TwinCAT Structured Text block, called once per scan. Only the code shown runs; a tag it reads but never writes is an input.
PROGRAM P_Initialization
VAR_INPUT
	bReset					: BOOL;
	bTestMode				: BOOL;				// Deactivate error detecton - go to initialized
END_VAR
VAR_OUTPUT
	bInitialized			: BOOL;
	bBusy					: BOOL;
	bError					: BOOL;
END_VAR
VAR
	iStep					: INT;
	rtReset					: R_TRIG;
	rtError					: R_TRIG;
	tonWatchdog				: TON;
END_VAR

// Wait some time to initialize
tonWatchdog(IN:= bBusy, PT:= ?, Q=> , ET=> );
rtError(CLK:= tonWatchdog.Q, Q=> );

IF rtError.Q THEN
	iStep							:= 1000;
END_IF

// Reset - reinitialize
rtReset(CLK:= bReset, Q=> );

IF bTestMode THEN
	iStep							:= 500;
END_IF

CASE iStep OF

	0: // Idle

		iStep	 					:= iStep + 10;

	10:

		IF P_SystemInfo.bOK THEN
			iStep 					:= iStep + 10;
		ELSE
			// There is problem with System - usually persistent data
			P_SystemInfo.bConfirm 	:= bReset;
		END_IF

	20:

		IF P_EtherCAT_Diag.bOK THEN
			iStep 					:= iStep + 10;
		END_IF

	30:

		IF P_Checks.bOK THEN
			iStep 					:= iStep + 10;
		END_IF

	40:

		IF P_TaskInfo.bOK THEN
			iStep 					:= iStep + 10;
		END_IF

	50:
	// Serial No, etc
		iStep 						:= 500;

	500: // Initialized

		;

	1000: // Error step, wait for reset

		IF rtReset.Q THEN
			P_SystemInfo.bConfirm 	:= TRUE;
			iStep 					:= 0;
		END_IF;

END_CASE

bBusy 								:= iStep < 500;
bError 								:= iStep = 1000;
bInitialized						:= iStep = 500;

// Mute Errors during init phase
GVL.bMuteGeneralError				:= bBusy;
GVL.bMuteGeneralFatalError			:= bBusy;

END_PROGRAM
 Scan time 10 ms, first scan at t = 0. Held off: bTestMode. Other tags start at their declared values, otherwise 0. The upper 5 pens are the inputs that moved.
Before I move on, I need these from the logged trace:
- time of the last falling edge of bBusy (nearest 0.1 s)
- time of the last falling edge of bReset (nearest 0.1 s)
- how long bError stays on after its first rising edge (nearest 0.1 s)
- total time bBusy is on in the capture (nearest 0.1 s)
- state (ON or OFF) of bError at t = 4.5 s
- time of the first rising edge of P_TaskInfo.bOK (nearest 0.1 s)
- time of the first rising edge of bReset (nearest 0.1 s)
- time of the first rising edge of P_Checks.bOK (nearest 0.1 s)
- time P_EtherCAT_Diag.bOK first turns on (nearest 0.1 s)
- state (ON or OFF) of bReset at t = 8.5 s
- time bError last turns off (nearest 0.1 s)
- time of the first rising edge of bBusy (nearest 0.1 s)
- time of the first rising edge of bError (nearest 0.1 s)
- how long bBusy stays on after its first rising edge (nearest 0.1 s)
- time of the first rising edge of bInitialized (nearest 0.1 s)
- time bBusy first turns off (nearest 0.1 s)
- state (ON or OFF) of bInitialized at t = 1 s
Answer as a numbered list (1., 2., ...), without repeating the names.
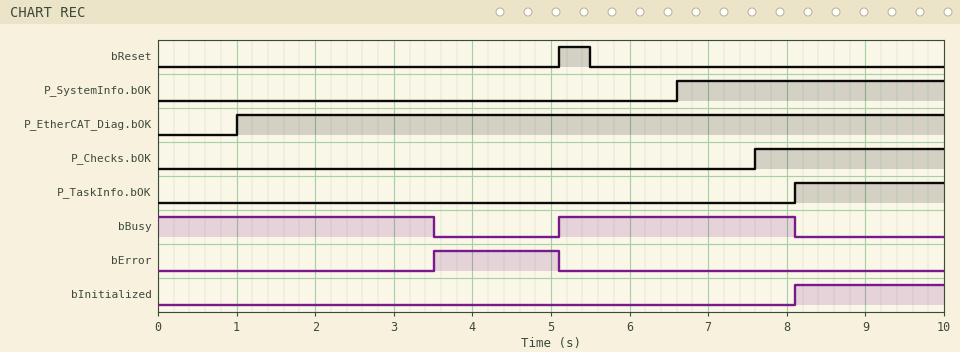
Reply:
1. 8.1 s
2. 5.5 s
3. 1.6 s
4. 6.5 s
5. ON
6. 8.1 s
7. 5.1 s
8. 7.6 s
9. 1.0 s
10. OFF
11. 5.1 s
12. 5.1 s
13. 3.5 s
14. 3.0 s
15. 8.1 s
16. 3.5 s
17. OFF
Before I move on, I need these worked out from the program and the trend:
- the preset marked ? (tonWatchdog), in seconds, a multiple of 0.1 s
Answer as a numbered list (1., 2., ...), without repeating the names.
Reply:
1. 3.5 s
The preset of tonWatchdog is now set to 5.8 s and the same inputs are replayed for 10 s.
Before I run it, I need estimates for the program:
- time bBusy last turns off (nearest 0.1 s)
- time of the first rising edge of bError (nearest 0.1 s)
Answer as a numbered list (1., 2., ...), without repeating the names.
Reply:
1. 5.8 s
2. 5.8 s
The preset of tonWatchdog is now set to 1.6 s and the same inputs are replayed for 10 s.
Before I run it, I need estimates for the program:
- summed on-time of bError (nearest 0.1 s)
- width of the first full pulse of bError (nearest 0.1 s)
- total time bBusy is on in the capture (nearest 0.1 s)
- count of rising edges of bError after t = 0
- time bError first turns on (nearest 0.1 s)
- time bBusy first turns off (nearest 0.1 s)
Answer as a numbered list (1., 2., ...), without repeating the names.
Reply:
1. 6.8 s
2. 3.5 s
3. 3.2 s
4. 2
5. 1.6 s
6. 1.6 s
